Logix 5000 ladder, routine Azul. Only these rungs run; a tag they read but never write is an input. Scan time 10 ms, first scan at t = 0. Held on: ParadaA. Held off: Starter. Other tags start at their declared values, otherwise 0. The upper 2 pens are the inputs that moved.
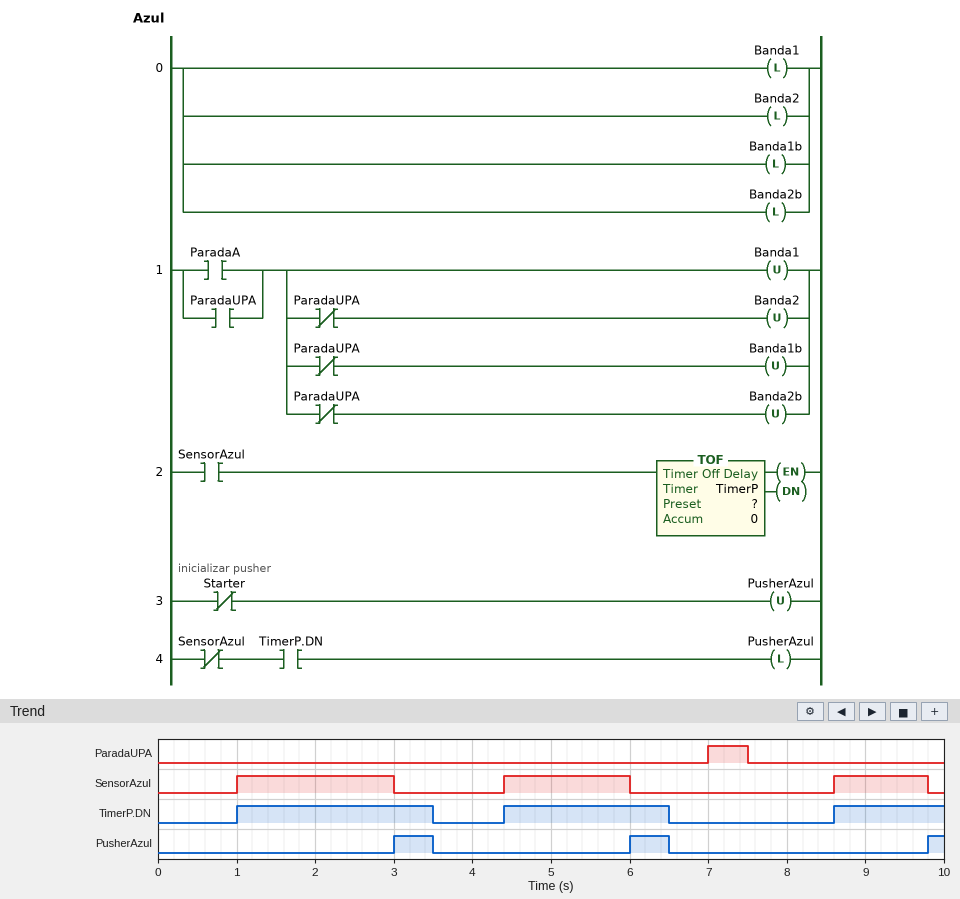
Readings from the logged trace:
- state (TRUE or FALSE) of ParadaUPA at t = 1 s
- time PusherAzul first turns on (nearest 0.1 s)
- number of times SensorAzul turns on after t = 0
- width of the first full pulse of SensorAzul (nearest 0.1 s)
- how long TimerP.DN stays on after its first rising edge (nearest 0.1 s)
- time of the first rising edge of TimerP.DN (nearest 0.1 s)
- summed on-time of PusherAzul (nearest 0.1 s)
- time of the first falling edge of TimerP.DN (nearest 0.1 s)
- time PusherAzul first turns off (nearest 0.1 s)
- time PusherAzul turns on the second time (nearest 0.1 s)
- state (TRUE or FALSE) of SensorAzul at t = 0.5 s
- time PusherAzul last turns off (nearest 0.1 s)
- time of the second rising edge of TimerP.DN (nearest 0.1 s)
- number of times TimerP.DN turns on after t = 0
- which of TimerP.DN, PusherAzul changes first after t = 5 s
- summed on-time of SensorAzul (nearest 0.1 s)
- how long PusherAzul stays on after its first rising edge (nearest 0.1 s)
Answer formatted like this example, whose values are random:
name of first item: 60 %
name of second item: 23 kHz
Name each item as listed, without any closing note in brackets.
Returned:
state (TRUE or FALSE) of ParadaUPA at t = 1 s: FALSE
time PusherAzul first turns on: 3.0 s
number of times SensorAzul turns on after t = 0: 3
width of the first full pulse of SensorAzul: 2.0 s
how long TimerP.DN stays on after its first rising edge: 2.5 s
time of the first rising edge of TimerP.DN: 1.0 s
summed on-time of PusherAzul: 1.2 s
time of the first falling edge of TimerP.DN: 3.5 s
time PusherAzul first turns off: 3.5 s
time PusherAzul turns on the second time: 6.0 s
state (TRUE or FALSE) of SensorAzul at t = 0.5 s: FALSE
time PusherAzul last turns off: 6.5 s
time of the second rising edge of TimerP.DN: 4.4 s
number of times TimerP.DN turns on after t = 0: 3
which of TimerP.DN, PusherAzul changes first after t = 5 s: PusherAzul
summed on-time of SensorAzul: 4.8 s
how long PusherAzul stays on after its first rising edge: 0.5 s
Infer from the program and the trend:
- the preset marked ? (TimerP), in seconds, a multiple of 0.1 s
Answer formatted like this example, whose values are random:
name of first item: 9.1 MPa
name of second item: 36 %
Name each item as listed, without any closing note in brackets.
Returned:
the preset marked ? (TimerP), in seconds, a multiple of 0.1 s: 0.5 s
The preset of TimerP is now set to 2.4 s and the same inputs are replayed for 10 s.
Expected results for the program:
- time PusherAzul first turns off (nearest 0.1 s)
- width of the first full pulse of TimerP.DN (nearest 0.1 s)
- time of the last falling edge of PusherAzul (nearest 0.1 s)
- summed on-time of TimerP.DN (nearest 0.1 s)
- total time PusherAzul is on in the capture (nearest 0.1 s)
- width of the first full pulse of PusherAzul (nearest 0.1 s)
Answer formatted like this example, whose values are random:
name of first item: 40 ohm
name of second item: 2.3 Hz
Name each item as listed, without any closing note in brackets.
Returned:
time PusherAzul first turns off: 4.4 s
width of the first full pulse of TimerP.DN: 7.4 s
time of the last falling edge of PusherAzul: 8.4 s
summed on-time of TimerP.DN: 8.8 s
total time PusherAzul is on in the capture: 4.0 s
width of the first full pulse of PusherAzul: 1.4 s
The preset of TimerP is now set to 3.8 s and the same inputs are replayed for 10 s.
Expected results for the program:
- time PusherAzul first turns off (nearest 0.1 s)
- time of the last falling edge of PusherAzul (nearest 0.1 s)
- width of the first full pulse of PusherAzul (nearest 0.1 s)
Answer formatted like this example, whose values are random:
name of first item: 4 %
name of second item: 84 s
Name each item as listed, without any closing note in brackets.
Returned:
time PusherAzul first turns off: 4.4 s
time of the last falling edge of PusherAzul: 8.6 s
width of the first full pulse of PusherAzul: 1.4 s
